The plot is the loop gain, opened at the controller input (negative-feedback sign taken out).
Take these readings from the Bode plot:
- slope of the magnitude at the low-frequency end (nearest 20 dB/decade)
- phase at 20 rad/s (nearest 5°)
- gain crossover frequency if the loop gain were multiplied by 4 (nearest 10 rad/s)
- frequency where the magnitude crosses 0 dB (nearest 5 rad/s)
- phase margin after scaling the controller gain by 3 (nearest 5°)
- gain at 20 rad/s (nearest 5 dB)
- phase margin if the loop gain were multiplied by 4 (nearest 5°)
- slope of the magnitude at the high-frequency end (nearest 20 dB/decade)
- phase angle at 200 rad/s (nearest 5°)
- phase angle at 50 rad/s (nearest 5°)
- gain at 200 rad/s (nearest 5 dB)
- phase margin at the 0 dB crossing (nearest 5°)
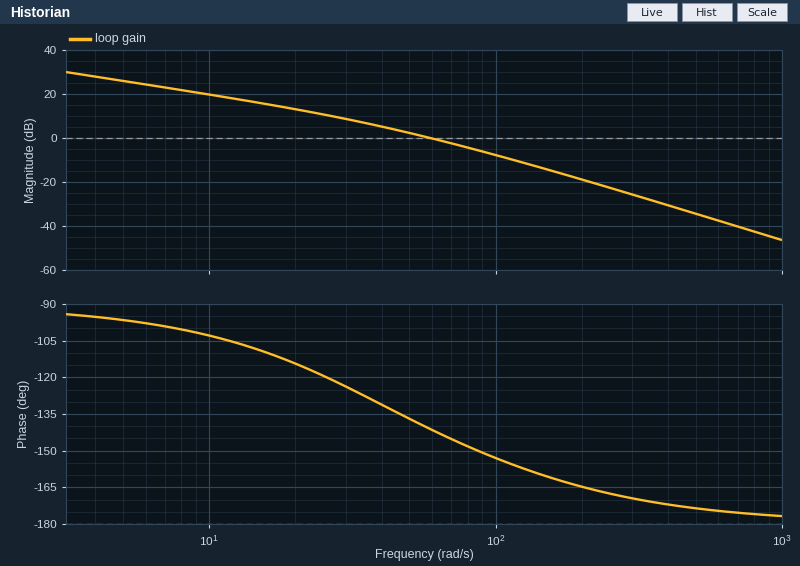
-20 dB/decade
-115°
130 rad/s
60 rad/s
25°
15 dB
20°
-40 dB/decade
-165°
-135°
-20 dB
40°
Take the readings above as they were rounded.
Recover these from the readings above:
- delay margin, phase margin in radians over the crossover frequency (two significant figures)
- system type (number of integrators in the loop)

0.012 s
1
